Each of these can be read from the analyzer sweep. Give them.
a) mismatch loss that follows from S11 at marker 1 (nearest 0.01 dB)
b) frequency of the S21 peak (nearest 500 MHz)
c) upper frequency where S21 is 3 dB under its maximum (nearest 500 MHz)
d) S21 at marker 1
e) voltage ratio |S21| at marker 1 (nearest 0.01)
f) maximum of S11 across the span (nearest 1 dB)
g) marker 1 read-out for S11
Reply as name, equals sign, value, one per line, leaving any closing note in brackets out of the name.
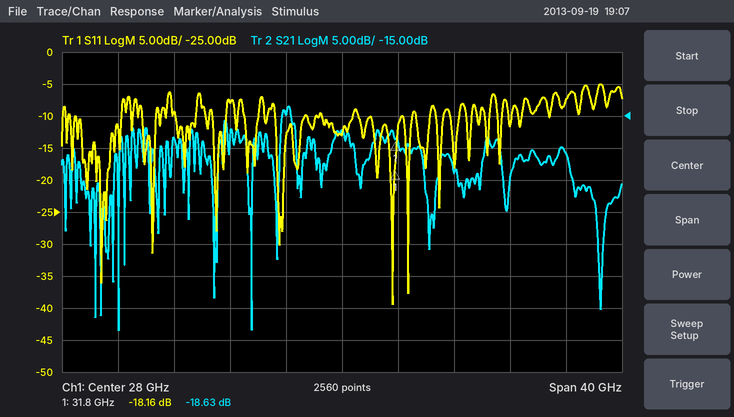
mismatch loss that follows from S11 at marker 1 = 0.07 dB
frequency of the S21 peak = 24.0 GHz
upper frequency where S21 is 3 dB under its maximum = 24.5 GHz
S21 at marker 1 = -18.63 dB
voltage ratio |S21| at marker 1 = 0.12
maximum of S11 across the span = -5 dB
marker 1 read-out for S11 = -18.16 dB
